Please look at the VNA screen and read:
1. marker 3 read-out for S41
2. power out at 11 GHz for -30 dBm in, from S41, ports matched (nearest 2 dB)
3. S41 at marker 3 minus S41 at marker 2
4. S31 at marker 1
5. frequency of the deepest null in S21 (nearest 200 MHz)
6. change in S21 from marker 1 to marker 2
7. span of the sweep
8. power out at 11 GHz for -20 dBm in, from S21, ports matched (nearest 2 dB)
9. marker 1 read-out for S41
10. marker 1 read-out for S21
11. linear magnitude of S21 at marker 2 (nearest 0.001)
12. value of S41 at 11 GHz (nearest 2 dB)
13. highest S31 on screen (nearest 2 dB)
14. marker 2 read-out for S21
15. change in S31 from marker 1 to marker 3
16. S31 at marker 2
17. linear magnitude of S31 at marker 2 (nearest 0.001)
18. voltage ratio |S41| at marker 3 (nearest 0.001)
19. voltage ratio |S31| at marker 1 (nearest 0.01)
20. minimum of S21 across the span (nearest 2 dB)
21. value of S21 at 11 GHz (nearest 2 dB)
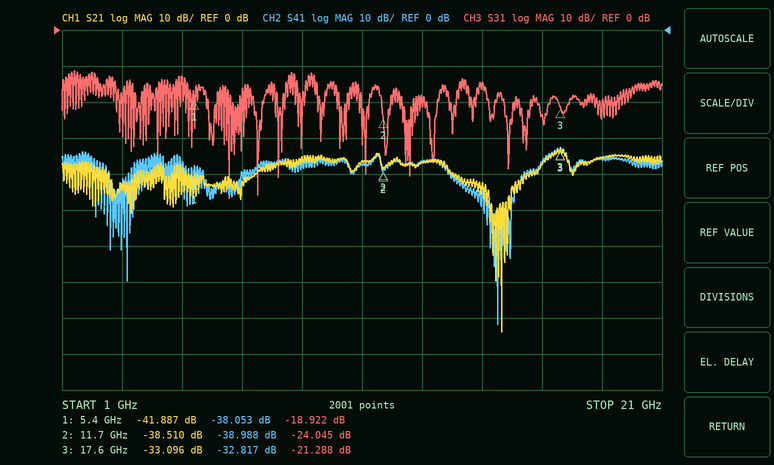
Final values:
-32.817 dB
-68 dBm
6.171 dB
-18.922 dB
15.6 GHz
3.377 dB
20 GHz
-56 dBm
-38.053 dB
-41.887 dB
0.012
-38 dB
-12 dB
-38.510 dB
-2.366 dB
-24.045 dB
0.063
0.023
0.11
-84 dB
-36 dB
